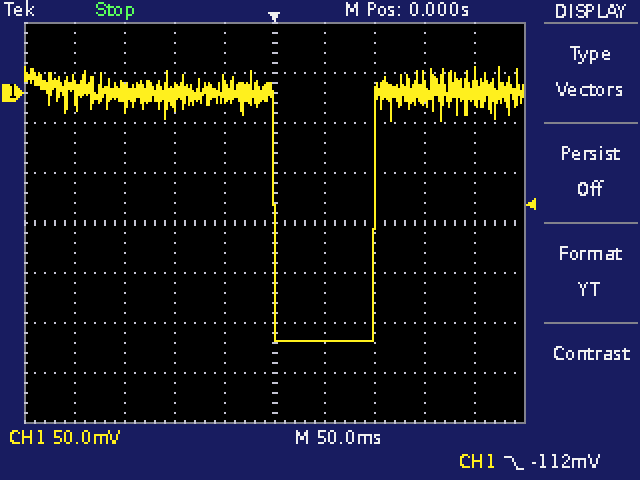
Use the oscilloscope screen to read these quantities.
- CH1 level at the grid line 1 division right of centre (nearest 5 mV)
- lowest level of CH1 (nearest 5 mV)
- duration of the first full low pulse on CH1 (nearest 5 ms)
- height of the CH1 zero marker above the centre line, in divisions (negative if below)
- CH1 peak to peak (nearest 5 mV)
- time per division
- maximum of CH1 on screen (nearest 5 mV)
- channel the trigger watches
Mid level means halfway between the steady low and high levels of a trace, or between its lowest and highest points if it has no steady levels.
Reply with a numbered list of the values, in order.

1. -250 mV
2. -250 mV
3. 100 ms
4. +2.6 div
5. 275 mV
6. 50 ms
7. 25 mV
8. CH1
